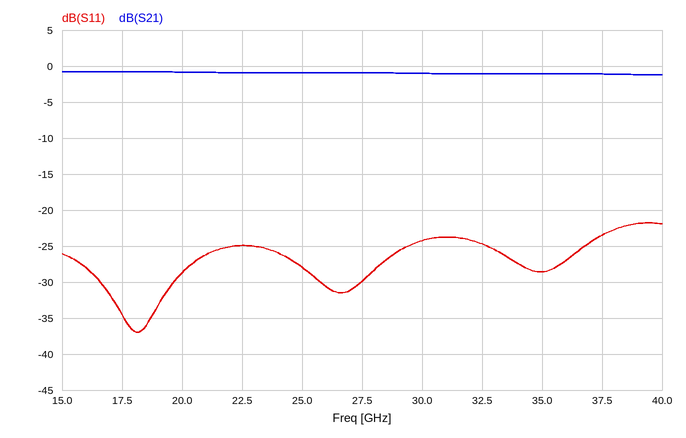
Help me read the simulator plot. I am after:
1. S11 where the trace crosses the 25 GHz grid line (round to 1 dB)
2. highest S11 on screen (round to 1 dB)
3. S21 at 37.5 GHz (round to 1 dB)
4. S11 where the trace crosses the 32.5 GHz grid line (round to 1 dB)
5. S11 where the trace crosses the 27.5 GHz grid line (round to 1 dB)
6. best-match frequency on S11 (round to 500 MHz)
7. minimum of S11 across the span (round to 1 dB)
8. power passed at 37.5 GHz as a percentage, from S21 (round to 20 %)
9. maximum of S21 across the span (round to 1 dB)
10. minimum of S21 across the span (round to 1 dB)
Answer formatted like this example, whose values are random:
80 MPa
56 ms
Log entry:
-28 dB
-22 dB
-1 dB
-25 dB
-30 dB
18.0 GHz
-37 dB
80 %
-1 dB
-1 dB
